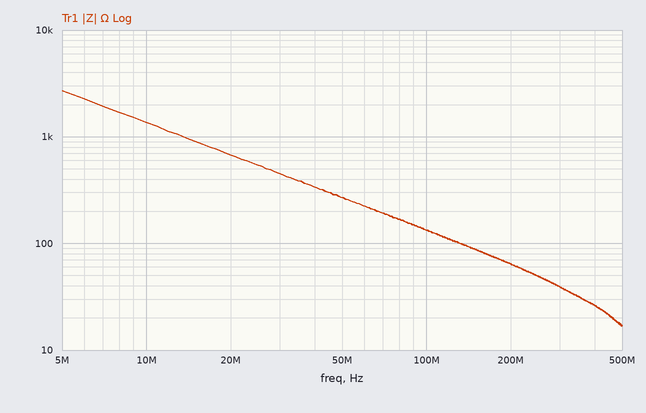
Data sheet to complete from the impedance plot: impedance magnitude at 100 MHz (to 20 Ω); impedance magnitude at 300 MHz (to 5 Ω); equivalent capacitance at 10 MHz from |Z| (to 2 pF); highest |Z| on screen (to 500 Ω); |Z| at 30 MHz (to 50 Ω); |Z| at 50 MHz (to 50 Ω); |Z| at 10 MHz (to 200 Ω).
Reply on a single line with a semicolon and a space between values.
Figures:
140 Ω; 40 Ω; 12 pF; 2.5 kΩ; 450 Ω; 250 Ω; 1.4 kΩ
